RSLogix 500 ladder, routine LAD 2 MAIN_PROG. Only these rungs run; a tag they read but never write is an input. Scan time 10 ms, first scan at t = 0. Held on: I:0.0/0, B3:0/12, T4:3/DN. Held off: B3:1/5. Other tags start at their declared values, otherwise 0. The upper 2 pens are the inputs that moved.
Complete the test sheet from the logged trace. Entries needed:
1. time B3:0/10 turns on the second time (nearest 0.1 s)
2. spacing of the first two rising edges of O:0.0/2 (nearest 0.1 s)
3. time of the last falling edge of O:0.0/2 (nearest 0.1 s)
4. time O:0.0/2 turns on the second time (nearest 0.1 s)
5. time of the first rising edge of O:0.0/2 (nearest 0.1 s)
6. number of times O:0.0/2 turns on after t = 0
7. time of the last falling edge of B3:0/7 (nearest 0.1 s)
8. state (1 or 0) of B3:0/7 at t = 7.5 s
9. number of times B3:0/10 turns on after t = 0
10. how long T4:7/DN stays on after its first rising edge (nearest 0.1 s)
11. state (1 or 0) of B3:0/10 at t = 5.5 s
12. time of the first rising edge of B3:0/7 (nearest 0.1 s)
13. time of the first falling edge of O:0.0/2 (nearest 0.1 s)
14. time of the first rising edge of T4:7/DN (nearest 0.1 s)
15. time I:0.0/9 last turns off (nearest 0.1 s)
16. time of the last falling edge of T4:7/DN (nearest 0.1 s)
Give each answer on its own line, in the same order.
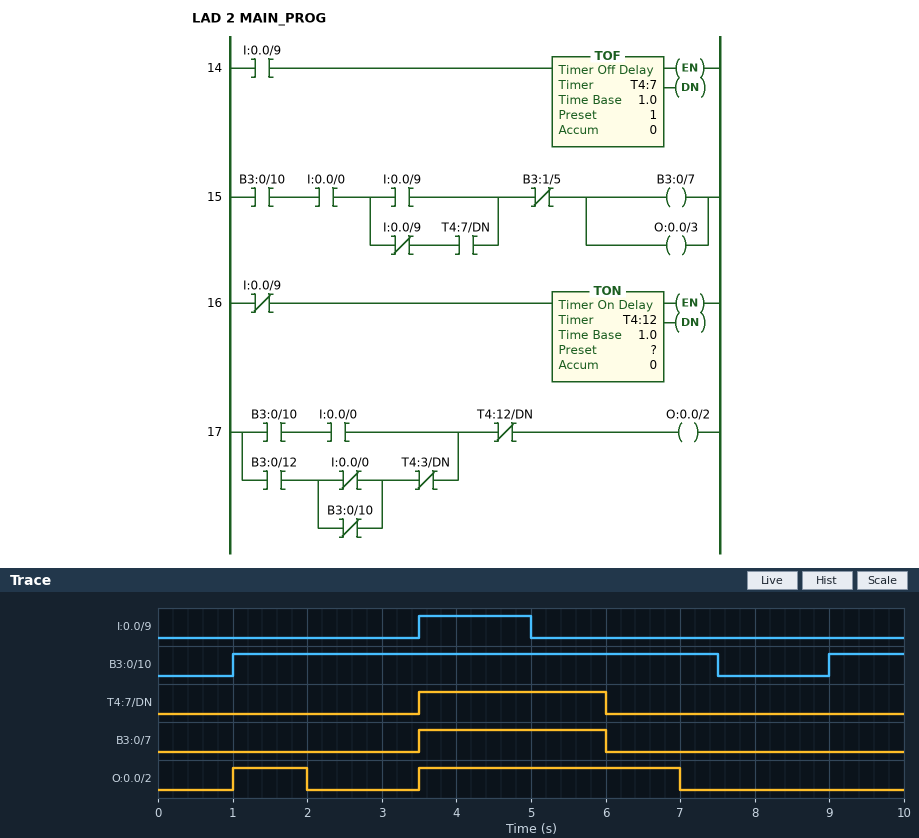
9.0 s
2.5 s
7.0 s
3.5 s
1.0 s
2
6.0 s
0
2
2.5 s
1
3.5 s
2.0 s
3.5 s
5.0 s
6.0 s
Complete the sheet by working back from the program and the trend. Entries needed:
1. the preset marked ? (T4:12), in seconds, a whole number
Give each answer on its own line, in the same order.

2 s
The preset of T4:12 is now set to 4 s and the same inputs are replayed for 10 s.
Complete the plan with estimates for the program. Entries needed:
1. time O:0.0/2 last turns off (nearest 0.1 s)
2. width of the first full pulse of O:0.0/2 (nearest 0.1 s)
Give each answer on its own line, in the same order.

7.5 s
6.5 s
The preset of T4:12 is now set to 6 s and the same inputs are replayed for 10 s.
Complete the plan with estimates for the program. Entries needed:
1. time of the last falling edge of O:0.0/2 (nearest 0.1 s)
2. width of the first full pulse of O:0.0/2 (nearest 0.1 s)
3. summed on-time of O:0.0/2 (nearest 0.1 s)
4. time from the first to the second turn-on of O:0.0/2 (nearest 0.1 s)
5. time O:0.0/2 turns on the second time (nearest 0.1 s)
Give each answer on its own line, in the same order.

7.5 s
6.5 s
7.5 s
8.0 s
9.0 s
